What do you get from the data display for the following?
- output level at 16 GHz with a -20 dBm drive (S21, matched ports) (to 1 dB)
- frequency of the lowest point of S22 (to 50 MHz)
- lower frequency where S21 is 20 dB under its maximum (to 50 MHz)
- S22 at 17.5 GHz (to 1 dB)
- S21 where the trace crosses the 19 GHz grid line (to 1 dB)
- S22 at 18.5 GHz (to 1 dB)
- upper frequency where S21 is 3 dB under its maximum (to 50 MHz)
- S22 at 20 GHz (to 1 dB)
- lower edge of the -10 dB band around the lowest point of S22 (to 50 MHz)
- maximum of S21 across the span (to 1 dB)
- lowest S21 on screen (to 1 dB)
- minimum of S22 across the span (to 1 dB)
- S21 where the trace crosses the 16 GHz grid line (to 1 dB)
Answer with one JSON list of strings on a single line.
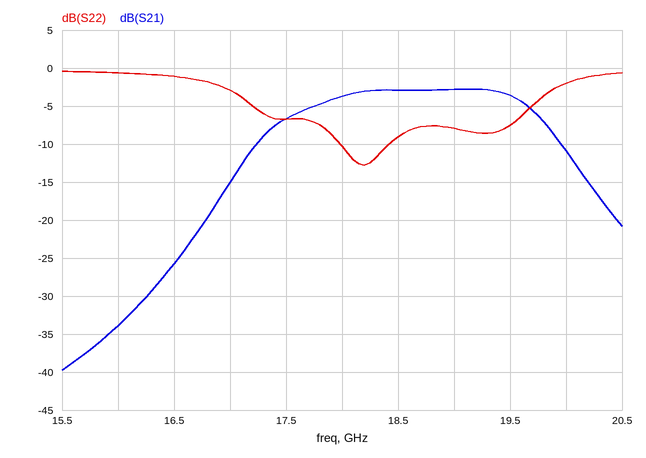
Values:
["-54 dBm", "18.20 GHz", "16.65 GHz", "-7 dB", "-3 dB", "-9 dB", "19.70 GHz", "-2 dB", "18.00 GHz", "-3 dB", "-40 dB", "-13 dB", "-34 dB"]
